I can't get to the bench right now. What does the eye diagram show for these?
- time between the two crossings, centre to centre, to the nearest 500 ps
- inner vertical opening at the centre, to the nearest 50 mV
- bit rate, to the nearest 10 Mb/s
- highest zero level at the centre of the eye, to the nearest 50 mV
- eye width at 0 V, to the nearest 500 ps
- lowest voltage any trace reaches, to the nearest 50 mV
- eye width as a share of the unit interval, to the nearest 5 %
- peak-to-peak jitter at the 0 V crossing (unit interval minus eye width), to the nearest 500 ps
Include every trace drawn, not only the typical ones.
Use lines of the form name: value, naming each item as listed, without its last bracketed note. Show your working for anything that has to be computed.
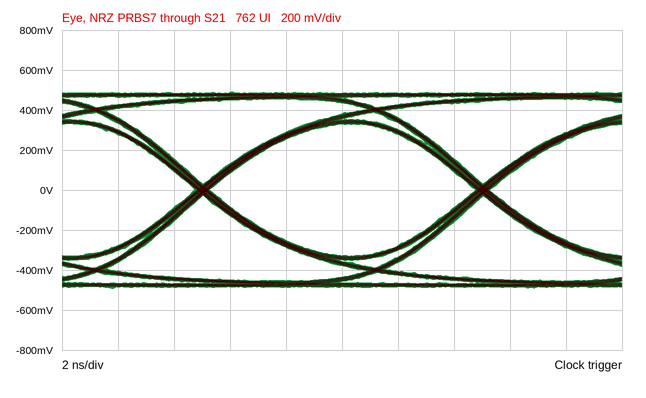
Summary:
time between the two crossings, centre to centre, to the nearest 500 ps: 10.0 ns
inner vertical opening at the centre, to the nearest 50 mV: 650 mV
bit rate, to the nearest 10 Mb/s: 100 Mb/s
highest zero level at the centre of the eye, to the nearest 50 mV: -350 mV
eye width at 0 V, to the nearest 500 ps: 9.5 ns
lowest voltage any trace reaches, to the nearest 50 mV: -500 mV
eye width as a share of the unit interval, to the nearest 5 %: 9.5 ns / 10.0 ns ≈ 95 %
peak-to-peak jitter at the 0 V crossing (unit interval minus eye width), to the nearest 500 ps: 500 ps
